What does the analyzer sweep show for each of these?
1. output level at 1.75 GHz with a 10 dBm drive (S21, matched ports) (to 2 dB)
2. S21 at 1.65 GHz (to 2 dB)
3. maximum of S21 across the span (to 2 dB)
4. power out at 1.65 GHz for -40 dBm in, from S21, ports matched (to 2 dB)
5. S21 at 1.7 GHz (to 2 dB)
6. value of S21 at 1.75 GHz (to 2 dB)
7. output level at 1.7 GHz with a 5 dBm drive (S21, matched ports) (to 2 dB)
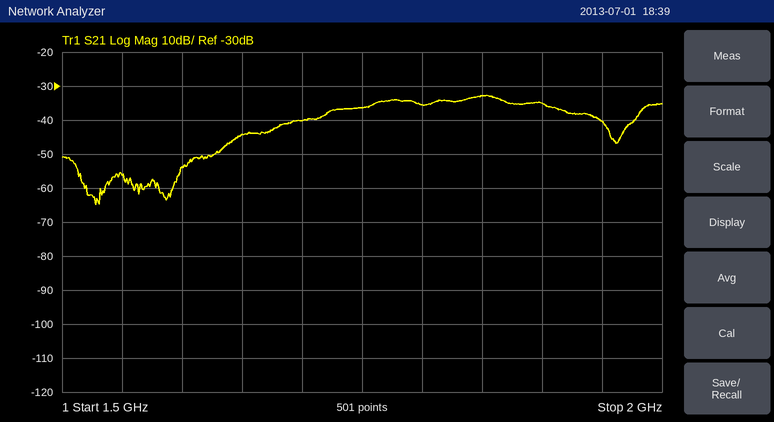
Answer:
-26 dBm
-44 dB
-32 dB
-84 dBm
-40 dB
-36 dB
-36 dBm
